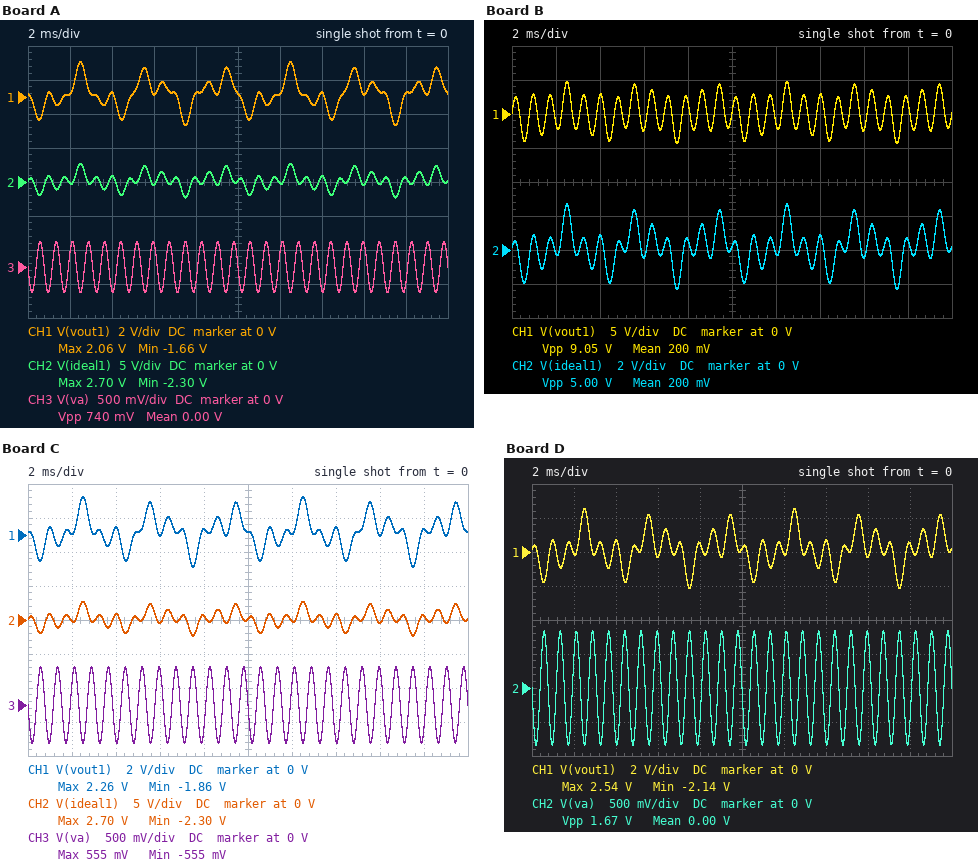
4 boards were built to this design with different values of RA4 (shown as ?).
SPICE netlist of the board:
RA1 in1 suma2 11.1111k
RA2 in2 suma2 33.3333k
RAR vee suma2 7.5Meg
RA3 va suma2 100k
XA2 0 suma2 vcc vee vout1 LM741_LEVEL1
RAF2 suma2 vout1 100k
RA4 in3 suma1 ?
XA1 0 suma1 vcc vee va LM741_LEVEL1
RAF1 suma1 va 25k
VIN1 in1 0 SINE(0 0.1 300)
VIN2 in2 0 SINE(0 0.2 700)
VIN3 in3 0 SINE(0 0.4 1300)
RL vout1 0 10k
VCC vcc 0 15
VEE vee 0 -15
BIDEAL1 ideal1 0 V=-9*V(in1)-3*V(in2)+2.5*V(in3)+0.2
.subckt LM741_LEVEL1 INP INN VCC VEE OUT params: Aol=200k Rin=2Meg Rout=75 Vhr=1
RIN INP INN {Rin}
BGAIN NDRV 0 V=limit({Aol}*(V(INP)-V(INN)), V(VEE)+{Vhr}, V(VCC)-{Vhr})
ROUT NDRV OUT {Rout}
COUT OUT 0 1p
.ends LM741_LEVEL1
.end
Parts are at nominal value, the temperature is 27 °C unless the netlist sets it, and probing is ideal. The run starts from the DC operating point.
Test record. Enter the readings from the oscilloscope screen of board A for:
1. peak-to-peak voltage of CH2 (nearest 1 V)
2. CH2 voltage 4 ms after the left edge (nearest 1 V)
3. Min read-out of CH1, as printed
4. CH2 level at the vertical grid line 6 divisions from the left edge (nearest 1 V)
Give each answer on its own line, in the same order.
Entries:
5 V
1 V
-1.66 V
0 V
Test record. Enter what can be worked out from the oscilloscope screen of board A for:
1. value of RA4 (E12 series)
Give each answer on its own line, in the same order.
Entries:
27 kΩ
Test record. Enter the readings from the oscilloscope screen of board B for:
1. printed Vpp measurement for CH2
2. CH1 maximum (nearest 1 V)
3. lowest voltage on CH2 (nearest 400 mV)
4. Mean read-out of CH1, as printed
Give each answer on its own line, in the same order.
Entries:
5.00 V
5 V
-2.4 V
200 mV
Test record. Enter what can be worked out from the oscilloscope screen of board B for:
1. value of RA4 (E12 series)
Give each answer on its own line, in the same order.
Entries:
3.3 kΩ
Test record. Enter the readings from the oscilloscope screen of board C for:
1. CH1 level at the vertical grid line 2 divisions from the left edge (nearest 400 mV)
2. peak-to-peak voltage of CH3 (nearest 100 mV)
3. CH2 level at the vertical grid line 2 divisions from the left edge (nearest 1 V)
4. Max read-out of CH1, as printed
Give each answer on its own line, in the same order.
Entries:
400 mV
1.1 V
1 V
2.26 V
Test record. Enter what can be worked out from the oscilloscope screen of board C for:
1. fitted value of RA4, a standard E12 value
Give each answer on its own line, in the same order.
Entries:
18 kΩ
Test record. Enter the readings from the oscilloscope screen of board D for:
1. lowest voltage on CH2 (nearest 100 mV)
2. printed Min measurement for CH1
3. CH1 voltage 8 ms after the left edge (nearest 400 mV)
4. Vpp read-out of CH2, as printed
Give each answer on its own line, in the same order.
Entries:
-800 mV
-2.14 V
400 mV
1.67 V
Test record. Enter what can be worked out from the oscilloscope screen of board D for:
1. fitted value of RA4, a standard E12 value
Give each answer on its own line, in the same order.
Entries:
12 kΩ
